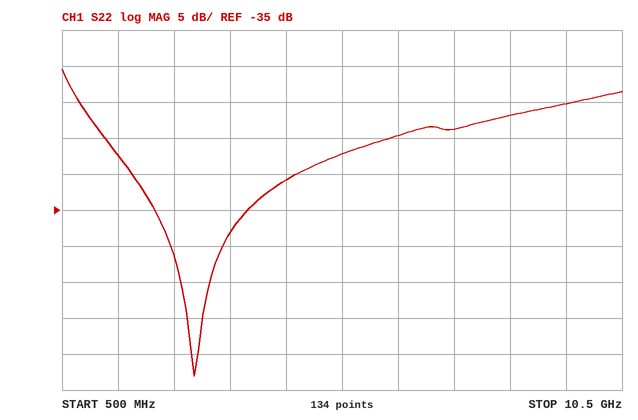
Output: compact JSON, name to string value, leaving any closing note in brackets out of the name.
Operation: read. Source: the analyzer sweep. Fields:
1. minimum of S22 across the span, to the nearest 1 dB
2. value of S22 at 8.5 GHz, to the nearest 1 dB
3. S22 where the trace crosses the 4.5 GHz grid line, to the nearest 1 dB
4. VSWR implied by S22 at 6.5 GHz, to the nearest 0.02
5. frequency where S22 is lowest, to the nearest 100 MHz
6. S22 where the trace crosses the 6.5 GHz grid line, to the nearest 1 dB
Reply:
{"minimum of S22 across the span, to the nearest 1 dB": "-58 dB", "value of S22 at 8.5 GHz, to the nearest 1 dB": "-22 dB", "S22 where the trace crosses the 4.5 GHz grid line, to the nearest 1 dB": "-31 dB", "VSWR implied by S22 at 6.5 GHz, to the nearest 0.02": "1.12", "frequency where S22 is lowest, to the nearest 100 MHz": "2.9 GHz", "S22 where the trace crosses the 6.5 GHz grid line, to the nearest 1 dB": "-25 dB"}
